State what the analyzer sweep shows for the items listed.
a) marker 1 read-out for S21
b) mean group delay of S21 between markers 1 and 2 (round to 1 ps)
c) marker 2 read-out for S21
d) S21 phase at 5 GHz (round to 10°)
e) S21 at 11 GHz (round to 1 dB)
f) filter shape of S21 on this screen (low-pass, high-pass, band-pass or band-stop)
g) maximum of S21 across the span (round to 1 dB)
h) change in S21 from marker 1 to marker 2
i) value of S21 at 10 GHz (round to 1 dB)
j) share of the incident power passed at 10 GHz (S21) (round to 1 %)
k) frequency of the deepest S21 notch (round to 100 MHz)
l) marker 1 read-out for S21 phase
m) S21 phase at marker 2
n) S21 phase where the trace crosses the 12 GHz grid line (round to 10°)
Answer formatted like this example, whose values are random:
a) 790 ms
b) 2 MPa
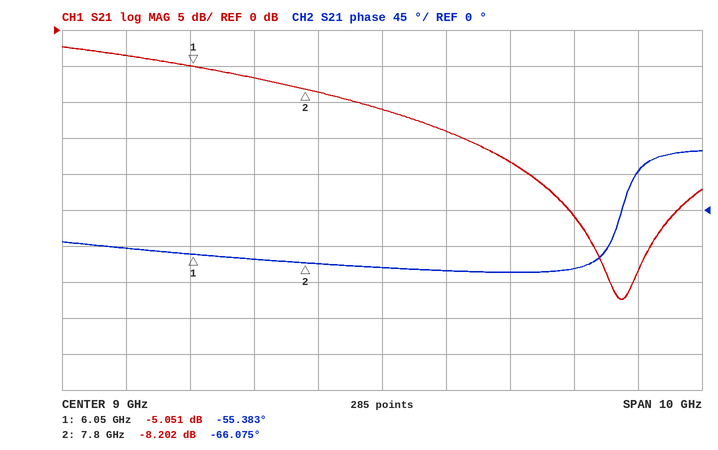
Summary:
a) -5.051 dB
b) 17 ps
c) -8.202 dB
d) -50°
e) -18 dB
f) low-pass
g) -2 dB
h) -3.151 dB
i) -14 dB
j) 4 %
k) 12.7 GHz
l) -55.383°
m) -66.075°
n) -70°
